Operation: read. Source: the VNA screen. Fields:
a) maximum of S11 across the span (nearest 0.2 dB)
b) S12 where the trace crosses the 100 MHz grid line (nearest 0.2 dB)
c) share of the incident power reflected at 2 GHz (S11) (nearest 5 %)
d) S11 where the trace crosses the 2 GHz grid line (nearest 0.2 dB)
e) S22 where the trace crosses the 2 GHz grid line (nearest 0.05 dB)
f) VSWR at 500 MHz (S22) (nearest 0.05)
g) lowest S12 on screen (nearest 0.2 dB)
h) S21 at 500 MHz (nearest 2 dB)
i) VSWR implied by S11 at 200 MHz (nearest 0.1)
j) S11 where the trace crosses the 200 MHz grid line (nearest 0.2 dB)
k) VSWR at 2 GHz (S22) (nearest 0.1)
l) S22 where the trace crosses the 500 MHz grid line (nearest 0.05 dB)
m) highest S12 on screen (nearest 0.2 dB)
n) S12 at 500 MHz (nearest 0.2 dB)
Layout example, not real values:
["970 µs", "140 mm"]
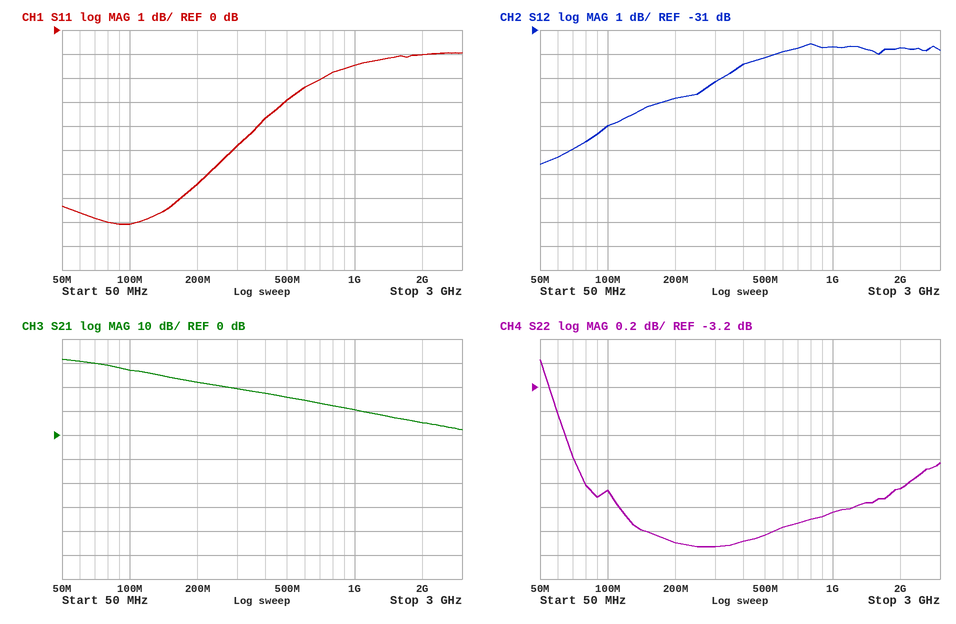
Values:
["-1.0 dB", "-35.0 dB", "80 %", "-1.0 dB", "-4.05 dB", "4.00", "-36.6 dB", "16 dB", "2.8", "-6.4 dB", "4.4", "-4.45 dB", "-31.6 dB", "-32.2 dB"]
